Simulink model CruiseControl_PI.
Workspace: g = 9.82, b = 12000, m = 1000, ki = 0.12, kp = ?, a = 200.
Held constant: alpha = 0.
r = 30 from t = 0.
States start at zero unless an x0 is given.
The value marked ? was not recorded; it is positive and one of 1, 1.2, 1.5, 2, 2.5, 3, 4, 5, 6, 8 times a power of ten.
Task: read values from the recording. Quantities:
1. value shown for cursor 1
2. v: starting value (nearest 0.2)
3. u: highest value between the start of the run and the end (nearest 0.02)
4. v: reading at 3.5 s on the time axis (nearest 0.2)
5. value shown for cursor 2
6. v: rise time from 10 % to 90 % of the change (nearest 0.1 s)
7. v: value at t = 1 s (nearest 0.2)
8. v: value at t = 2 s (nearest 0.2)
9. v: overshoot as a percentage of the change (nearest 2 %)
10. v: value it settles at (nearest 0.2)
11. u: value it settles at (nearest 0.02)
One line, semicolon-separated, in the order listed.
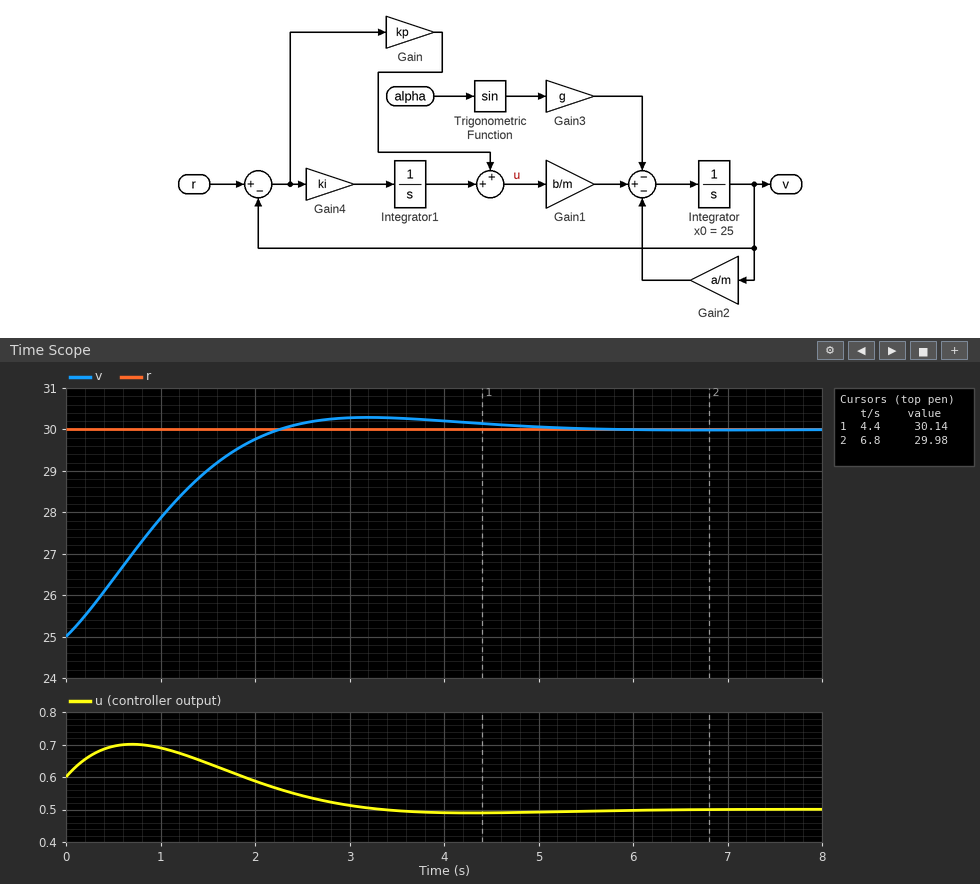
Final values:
30.14; 25.0; 0.70; 30.2; 29.98; 1.6 s; 27.8; 29.8; 6 %; 30.0; 0.50
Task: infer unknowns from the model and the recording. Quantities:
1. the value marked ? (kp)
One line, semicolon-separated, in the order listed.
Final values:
0.12
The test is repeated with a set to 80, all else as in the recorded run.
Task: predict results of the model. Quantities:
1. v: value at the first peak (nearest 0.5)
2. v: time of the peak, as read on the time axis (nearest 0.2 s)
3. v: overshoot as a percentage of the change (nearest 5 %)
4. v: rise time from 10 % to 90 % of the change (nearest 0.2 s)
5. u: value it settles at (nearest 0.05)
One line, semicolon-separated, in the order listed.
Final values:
30.5; 2.4 s; 15 %; 1.0 s; 0.20
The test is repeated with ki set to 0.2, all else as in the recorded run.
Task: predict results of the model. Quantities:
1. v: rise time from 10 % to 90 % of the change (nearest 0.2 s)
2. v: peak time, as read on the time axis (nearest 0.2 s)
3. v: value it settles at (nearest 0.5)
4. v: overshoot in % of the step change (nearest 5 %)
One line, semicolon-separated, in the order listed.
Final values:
1.0 s; 2.2 s; 30.0; 15 %
